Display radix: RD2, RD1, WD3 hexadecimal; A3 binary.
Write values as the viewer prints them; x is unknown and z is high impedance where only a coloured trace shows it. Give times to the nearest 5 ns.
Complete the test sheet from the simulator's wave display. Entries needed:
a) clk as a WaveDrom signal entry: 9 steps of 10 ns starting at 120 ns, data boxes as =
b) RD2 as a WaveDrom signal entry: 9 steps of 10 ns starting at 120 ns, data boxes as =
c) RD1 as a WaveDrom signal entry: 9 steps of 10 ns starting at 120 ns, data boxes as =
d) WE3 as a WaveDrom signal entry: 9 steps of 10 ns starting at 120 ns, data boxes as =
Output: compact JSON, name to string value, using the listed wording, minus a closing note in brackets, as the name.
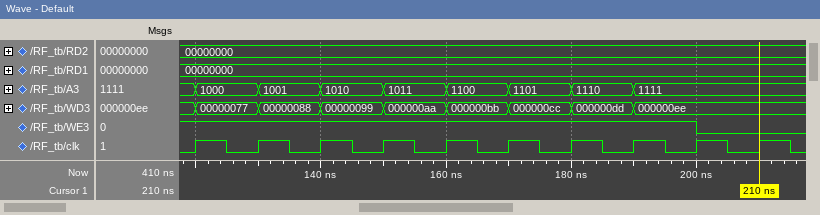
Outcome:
{"clk as a WaveDrom signal entry: 9 steps of 10 ns starting at 120 ns, data boxes as =": "{name: 'clk', wave: 'p........'}", "RD2 as a WaveDrom signal entry: 9 steps of 10 ns starting at 120 ns, data boxes as =": "{name: 'RD2', wave: '=........', data: '00000000'}", "RD1 as a WaveDrom signal entry: 9 steps of 10 ns starting at 120 ns, data boxes as =": "{name: 'RD1', wave: '=........', data: '00000000'}", "WE3 as a WaveDrom signal entry: 9 steps of 10 ns starting at 120 ns, data boxes as =": "{name: 'WE3', wave: '1.......0'}"}
